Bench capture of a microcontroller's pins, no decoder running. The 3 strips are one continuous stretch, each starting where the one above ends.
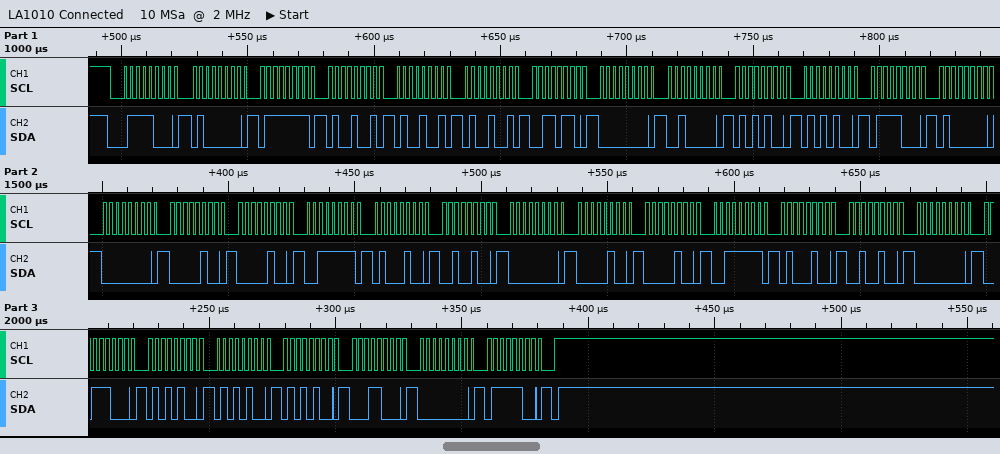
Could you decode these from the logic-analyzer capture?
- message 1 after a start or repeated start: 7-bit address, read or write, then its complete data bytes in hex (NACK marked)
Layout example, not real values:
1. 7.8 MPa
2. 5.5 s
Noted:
1. 0x3C write: 40 7F 49 49 49 36 00 20 54 54 78 40 00 04 04 3F 44 24 00 04 04 3F 44 24 00 38 54 54 54 18 00 7C
